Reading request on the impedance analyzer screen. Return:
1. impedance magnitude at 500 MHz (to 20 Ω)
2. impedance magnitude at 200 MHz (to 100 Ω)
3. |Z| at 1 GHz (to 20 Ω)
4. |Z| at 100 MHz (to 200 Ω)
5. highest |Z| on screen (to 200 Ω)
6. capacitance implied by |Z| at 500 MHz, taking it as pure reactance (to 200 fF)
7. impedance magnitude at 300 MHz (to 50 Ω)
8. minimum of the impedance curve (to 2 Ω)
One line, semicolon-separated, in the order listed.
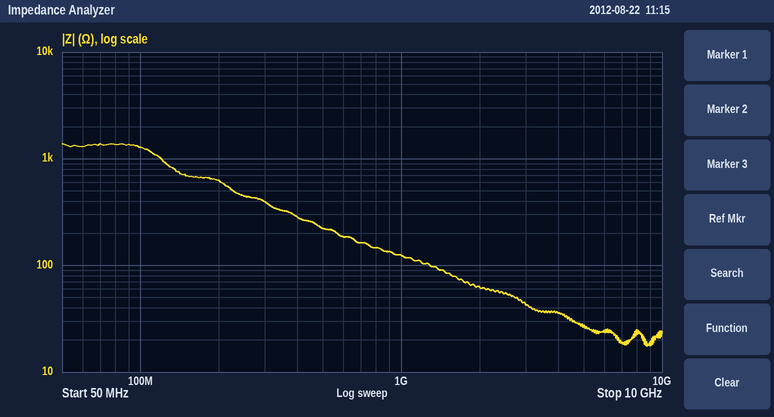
220 Ω; 600 Ω; 120 Ω; 1.2 kΩ; 1.4 kΩ; 1.4 pF; 400 Ω; 18 Ω
